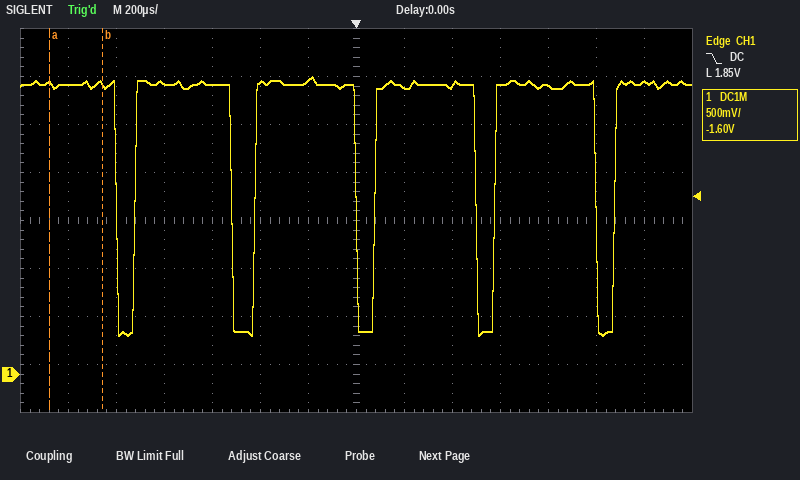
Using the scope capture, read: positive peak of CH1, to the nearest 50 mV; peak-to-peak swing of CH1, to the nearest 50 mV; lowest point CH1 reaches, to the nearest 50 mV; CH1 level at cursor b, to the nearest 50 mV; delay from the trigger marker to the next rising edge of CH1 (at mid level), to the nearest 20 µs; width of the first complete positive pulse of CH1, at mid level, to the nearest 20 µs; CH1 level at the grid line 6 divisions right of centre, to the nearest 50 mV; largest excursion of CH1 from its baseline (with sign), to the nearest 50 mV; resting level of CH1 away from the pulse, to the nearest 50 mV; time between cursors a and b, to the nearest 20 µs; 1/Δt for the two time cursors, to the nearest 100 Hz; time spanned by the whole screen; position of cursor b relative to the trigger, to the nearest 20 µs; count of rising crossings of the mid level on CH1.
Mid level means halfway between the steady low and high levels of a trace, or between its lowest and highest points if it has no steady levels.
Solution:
3.10 V
2.70 V
400 mV
3.00 V
80 µs
400 µs
3.05 V
-2.60 V
3.00 V
220 µs
4.5 kHz
2.8 ms
-1.06 ms
5
